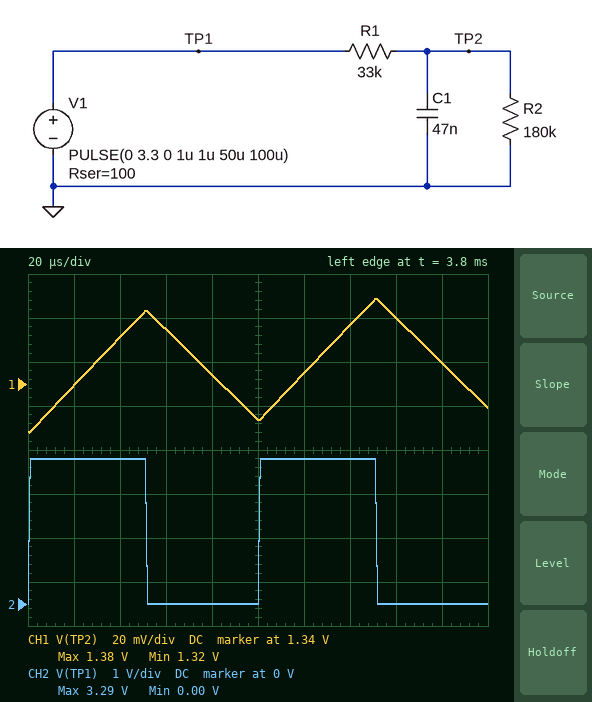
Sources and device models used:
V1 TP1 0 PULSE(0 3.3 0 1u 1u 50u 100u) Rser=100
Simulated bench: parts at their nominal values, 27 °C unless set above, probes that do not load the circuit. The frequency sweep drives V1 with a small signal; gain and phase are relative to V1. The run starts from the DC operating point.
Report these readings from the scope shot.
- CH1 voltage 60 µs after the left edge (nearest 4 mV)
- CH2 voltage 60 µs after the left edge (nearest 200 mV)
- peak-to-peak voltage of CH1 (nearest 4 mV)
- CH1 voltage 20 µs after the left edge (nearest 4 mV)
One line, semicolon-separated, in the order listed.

1.364 V; 0 V; 60 mV; 1.340 V
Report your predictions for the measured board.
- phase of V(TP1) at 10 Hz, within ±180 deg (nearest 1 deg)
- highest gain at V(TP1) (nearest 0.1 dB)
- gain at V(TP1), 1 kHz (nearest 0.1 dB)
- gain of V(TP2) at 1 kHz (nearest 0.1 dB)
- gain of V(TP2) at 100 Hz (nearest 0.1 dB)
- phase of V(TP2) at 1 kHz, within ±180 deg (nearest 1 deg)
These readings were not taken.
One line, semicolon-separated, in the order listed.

0 deg; 0 dB; 0 dB; -19.9 dB; -3.7 dB; -83 deg
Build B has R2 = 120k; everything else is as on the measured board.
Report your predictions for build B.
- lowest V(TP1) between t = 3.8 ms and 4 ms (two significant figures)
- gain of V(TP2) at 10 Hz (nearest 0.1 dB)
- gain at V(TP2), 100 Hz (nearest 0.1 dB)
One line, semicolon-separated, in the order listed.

3.7 mV; -2.1 dB; -4.1 dB
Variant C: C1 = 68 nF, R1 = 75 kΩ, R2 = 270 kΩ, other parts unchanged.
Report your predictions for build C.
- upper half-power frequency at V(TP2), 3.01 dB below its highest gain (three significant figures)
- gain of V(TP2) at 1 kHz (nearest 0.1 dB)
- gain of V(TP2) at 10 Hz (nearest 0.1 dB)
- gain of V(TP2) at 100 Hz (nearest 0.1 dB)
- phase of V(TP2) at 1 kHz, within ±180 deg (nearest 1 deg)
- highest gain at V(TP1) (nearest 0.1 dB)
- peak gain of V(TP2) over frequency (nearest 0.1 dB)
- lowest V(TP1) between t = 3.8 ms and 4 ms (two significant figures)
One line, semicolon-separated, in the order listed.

39.8 Hz; -30.1 dB; -2.4 dB; -10.8 dB; -88 deg; 0 dB; -2.1 dB; 1.1 mV
